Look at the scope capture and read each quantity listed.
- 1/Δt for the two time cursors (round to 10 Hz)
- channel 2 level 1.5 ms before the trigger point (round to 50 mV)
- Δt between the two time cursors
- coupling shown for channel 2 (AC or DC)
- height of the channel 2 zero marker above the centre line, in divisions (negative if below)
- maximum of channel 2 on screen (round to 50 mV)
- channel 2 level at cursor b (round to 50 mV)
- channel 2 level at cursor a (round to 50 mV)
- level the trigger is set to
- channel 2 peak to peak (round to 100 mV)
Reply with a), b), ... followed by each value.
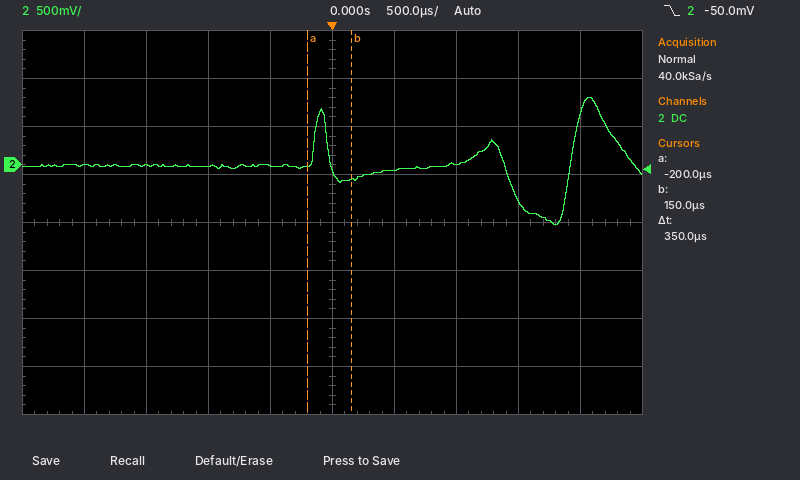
a) 2.86 kHz
b) 0 mV
c) 350 µs
d) DC
e) +1.2 div
f) 700 mV
g) -150 mV
h) 0 mV
i) -50.0 mV
j) 1.30 V
